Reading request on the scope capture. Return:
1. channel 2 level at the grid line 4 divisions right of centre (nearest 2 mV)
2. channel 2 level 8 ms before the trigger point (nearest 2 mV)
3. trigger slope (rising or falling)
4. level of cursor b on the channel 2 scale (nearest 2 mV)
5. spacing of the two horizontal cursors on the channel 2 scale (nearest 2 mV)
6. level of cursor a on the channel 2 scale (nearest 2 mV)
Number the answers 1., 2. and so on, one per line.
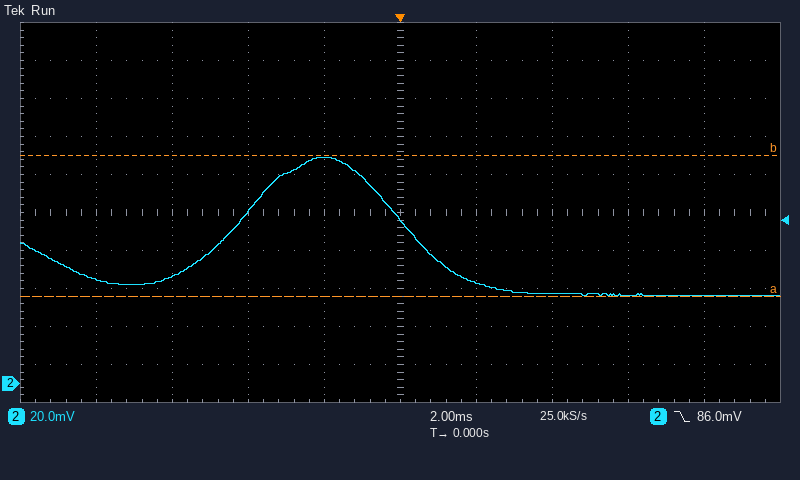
1. 46 mV
2. 54 mV
3. falling
4. 120 mV
5. 74 mV
6. 46 mV
